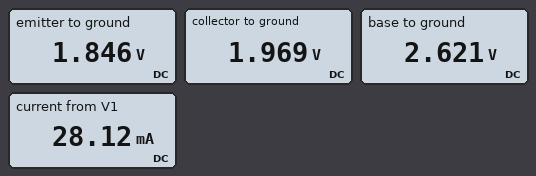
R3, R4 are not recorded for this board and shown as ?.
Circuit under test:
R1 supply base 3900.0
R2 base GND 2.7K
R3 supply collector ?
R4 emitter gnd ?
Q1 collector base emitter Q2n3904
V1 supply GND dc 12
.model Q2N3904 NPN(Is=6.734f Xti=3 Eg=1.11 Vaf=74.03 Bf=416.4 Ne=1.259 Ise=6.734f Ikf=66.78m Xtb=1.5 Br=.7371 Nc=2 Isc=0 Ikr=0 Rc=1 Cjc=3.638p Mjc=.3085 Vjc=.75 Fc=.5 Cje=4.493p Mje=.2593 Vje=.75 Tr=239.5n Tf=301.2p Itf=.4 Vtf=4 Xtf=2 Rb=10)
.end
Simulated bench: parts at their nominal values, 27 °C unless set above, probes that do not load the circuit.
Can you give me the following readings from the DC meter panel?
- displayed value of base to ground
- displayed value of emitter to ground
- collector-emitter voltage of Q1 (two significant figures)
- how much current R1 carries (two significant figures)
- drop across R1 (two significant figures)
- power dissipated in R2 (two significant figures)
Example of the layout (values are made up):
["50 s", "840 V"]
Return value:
["2.621 V", "1.846 V", "120 mV", "2.4 mA", "9.4 V", "2.5 mW"]
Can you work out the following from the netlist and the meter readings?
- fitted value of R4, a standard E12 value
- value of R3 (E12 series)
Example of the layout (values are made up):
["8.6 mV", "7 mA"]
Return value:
["68 Ω", "390 Ω"]
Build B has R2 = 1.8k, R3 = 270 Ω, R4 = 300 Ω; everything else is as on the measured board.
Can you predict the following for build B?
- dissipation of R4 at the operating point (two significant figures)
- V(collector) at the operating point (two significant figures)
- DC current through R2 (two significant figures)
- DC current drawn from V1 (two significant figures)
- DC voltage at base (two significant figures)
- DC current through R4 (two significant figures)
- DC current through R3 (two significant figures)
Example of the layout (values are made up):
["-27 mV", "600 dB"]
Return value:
["30 mW", "9.3 V", "2.1 mA", "12 mA", "3.7 V", "10 mA", "9.9 mA"]
